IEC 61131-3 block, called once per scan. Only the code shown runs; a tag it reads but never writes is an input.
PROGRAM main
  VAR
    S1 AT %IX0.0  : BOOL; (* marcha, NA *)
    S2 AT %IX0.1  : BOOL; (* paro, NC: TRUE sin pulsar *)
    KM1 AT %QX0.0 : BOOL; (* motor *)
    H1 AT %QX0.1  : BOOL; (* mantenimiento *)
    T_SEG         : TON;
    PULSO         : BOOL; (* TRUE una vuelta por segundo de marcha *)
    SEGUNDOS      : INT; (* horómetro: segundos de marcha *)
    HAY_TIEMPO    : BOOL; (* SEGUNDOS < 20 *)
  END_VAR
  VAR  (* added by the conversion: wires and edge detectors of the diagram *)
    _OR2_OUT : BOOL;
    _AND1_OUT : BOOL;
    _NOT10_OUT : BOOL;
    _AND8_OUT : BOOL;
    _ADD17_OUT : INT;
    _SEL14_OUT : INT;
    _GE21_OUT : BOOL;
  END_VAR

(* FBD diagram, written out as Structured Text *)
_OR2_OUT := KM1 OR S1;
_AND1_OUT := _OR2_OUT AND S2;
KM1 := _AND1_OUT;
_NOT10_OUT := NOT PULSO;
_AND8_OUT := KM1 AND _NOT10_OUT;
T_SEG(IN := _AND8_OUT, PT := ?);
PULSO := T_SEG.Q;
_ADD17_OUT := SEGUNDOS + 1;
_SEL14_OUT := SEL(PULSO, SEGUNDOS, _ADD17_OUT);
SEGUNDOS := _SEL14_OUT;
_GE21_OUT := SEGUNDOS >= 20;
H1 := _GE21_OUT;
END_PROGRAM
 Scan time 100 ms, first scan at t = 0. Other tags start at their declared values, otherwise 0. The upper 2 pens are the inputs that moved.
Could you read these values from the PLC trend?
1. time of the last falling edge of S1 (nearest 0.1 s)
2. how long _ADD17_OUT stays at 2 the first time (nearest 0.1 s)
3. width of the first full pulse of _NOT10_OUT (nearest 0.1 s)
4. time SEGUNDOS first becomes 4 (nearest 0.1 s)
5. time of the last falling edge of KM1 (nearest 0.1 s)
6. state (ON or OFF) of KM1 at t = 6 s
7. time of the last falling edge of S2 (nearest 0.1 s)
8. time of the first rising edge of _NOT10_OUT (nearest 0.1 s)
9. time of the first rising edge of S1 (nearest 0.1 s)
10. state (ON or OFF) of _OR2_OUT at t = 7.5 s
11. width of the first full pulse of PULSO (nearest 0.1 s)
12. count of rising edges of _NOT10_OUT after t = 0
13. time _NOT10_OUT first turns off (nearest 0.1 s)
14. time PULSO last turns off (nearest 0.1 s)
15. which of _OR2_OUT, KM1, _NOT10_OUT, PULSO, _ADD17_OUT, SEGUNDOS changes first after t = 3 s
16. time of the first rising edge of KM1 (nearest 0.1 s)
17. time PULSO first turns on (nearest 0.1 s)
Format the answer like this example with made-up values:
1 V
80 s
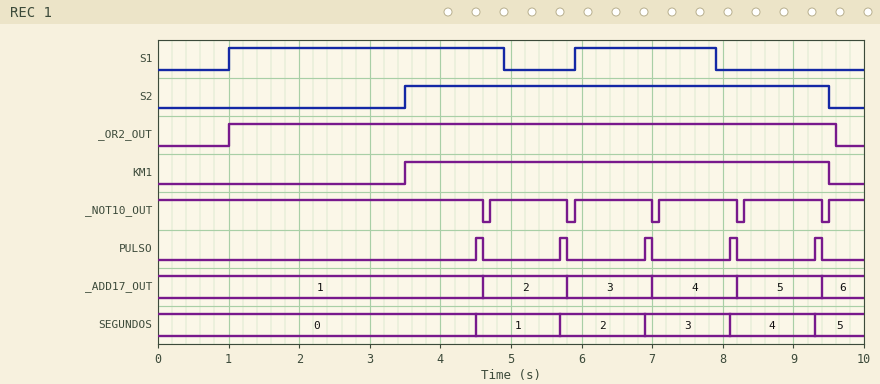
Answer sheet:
7.9 s
1.2 s
1.1 s
8.1 s
9.5 s
ON
9.5 s
4.7 s
1.0 s
ON
0.1 s
5
4.6 s
9.4 s
KM1
3.5 s
4.5 s
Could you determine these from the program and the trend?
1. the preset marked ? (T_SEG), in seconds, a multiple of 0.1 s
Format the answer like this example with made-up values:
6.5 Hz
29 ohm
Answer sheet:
1.0 s
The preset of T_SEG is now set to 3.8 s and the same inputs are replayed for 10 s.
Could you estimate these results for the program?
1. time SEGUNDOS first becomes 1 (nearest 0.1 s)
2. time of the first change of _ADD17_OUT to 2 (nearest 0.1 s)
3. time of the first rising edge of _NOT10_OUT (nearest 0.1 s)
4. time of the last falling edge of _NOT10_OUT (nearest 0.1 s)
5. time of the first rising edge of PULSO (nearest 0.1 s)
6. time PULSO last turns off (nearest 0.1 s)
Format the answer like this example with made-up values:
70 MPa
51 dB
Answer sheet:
7.3 s
7.4 s
7.5 s
7.4 s
7.3 s
7.4 s
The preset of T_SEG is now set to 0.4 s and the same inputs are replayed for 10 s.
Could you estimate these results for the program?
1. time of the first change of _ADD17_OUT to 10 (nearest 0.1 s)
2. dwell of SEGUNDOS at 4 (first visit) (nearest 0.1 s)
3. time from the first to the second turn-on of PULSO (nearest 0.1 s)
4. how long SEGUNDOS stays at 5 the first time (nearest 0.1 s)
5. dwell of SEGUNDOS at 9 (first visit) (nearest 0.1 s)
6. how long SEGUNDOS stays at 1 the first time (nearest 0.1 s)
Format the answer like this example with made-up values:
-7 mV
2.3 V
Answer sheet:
8.8 s
0.6 s
0.6 s
0.6 s
0.6 s
0.6 s
